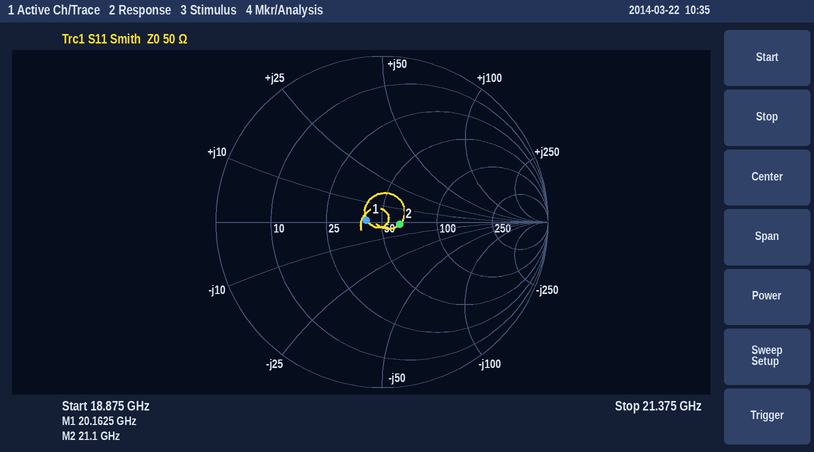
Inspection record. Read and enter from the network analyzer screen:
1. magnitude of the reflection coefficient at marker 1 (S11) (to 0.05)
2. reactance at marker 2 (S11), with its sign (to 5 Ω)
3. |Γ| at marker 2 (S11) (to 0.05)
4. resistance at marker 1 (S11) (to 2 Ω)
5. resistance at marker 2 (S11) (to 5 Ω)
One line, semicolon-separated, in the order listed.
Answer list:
0.10; 0 Ω; 0.10; 42 Ω; 60 Ω
